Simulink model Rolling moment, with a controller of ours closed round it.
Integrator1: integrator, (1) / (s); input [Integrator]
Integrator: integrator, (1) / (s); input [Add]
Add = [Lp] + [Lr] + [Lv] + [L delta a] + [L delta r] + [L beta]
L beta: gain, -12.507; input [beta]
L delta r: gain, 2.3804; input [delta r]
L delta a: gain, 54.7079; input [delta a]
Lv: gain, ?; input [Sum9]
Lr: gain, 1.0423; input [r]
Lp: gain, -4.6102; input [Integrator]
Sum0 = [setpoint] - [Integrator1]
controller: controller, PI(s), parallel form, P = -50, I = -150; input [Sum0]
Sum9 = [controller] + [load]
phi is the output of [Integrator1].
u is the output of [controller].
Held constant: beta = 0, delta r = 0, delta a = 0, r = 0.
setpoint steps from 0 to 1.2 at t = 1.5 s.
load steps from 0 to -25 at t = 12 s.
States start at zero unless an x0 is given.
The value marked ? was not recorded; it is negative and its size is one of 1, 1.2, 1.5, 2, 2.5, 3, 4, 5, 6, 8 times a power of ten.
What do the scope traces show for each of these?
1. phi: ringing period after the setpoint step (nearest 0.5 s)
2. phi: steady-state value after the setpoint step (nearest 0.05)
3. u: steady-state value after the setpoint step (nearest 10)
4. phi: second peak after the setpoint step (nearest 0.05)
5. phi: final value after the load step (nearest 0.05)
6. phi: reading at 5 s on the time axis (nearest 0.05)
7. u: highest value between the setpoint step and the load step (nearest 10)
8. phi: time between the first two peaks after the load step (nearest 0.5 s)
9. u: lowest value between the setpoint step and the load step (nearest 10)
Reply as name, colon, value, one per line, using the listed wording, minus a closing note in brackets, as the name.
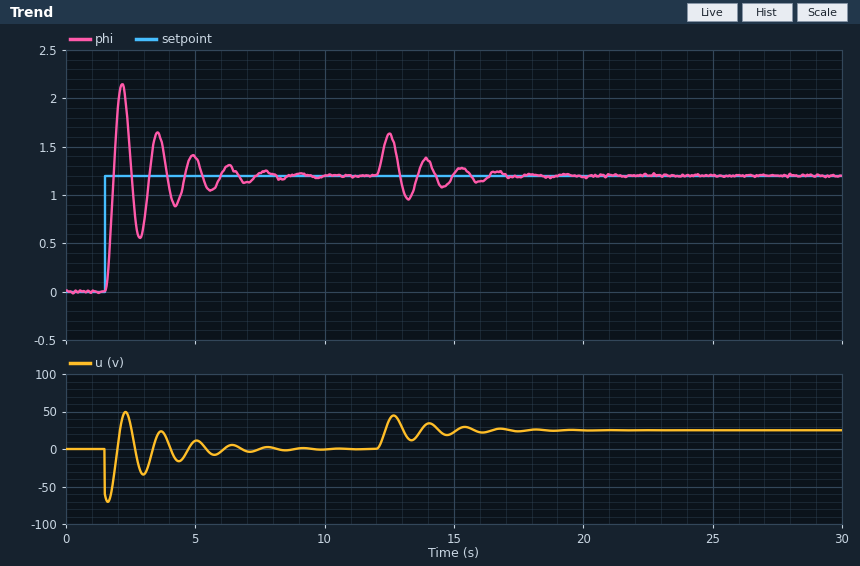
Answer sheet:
phi: ringing period after the setpoint step: 1.5 s
phi: steady-state value after the setpoint step: 1.20
u: steady-state value after the setpoint step: 0
phi: second peak after the setpoint step: 1.65
phi: final value after the load step: 1.20
phi: reading at 5 s on the time axis: 1.40
u: highest value between the setpoint step and the load step: 50
phi: time between the first two peaks after the load step: 1.5 s
u: lowest value between the setpoint step and the load step: -70
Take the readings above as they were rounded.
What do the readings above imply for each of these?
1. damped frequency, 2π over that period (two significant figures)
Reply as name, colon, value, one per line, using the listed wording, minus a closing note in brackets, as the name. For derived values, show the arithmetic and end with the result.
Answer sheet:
damped frequency, 2π over that period: 2π / 1.5 = 4.2 rad/s
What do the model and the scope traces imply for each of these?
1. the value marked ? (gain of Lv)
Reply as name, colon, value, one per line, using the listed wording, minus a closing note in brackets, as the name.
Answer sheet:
the value marked ?: -0.5
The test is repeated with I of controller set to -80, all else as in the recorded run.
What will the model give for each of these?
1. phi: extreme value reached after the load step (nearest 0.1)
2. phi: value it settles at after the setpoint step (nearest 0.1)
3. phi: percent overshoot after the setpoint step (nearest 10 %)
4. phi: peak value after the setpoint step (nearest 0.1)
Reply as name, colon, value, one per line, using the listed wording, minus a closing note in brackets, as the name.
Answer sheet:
phi: extreme value reached after the load step: 1.7
phi: value it settles at after the setpoint step: 1.2
phi: percent overshoot after the setpoint step: 60 %
phi: peak value after the setpoint step: 1.9
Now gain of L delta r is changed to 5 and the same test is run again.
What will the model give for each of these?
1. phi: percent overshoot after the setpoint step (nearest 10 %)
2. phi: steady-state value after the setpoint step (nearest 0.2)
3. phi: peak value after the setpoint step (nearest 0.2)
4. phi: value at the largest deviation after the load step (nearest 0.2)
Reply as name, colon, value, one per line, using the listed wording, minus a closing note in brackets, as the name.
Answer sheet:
phi: percent overshoot after the setpoint step: 80 %
phi: steady-state value after the setpoint step: 1.2
phi: peak value after the setpoint step: 2.2
phi: value at the largest deviation after the load step: 1.6
